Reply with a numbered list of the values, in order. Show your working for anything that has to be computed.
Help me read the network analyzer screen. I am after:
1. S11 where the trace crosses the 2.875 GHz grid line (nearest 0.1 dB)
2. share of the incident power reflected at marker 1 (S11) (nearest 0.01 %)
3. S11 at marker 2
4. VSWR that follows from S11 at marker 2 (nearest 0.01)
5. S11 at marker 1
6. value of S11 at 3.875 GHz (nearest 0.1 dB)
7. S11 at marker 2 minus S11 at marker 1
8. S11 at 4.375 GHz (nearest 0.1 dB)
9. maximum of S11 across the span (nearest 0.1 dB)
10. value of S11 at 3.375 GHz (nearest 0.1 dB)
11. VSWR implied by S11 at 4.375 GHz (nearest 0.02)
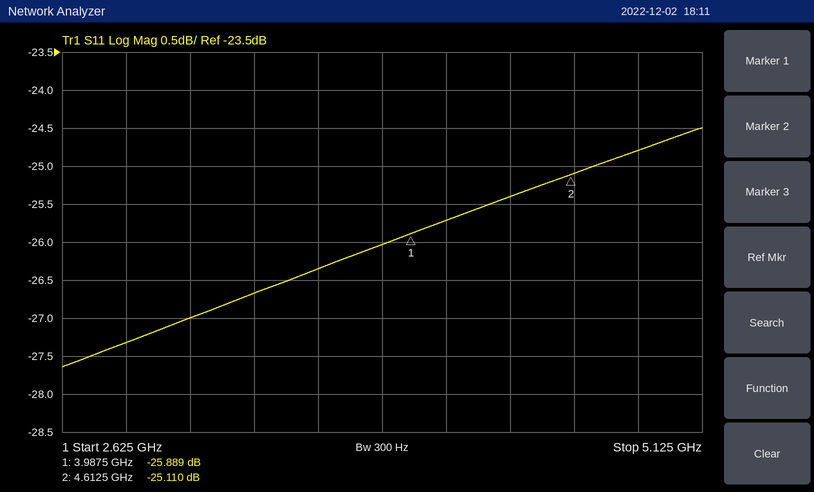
1. -27.3 dB
2. 10^(-25.889/10) ≈ 0.26 %
3. -25.110 dB
4. (1 + 0.0555)/(1 − 0.0555) ≈ 1.12
5. -25.889 dB
6. -26.0 dB
7. -25.11 − (-25.889) = 0.779 dB
8. -25.4 dB
9. -24.5 dB
10. -26.7 dB
11. |Γ| = 10^(-25.4/20) = 0.0537; VSWR = (1 + 0.0537)/(1 − 0.0537) ≈ 1.11, so 1.12 to the nearest 0.02
